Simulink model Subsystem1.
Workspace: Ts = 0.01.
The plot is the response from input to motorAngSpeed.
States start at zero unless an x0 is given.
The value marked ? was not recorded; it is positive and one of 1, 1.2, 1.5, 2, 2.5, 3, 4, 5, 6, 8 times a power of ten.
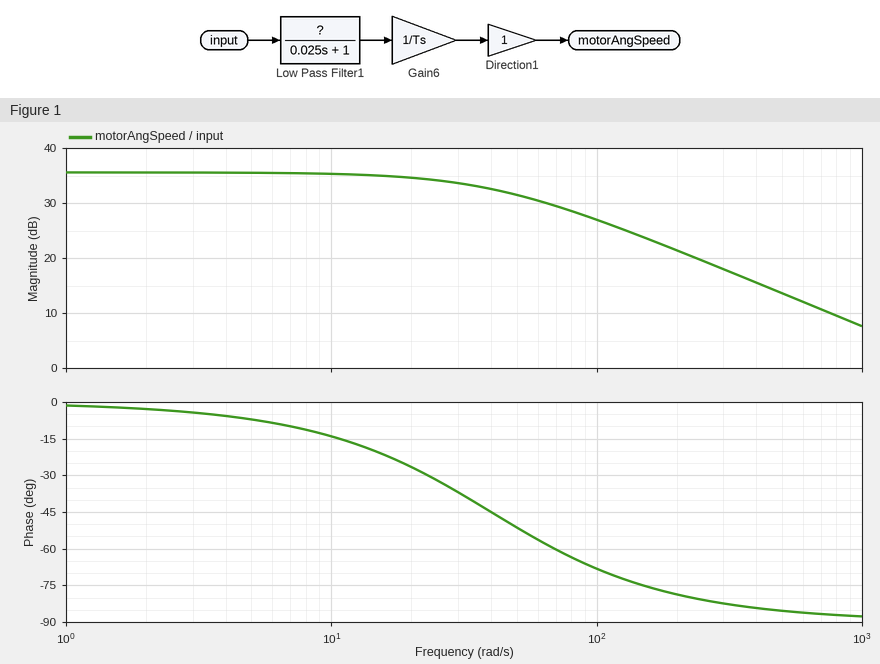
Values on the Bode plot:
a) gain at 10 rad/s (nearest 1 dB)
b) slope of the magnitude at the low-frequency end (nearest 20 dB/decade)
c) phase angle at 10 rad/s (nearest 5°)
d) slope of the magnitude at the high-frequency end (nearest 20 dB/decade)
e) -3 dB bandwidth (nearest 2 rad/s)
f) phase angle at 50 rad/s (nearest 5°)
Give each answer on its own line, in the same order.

35 dB
0 dB/decade
-15°
-20 dB/decade
40 rad/s
-50°
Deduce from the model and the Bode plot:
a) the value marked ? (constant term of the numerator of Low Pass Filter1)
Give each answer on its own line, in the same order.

0.6
